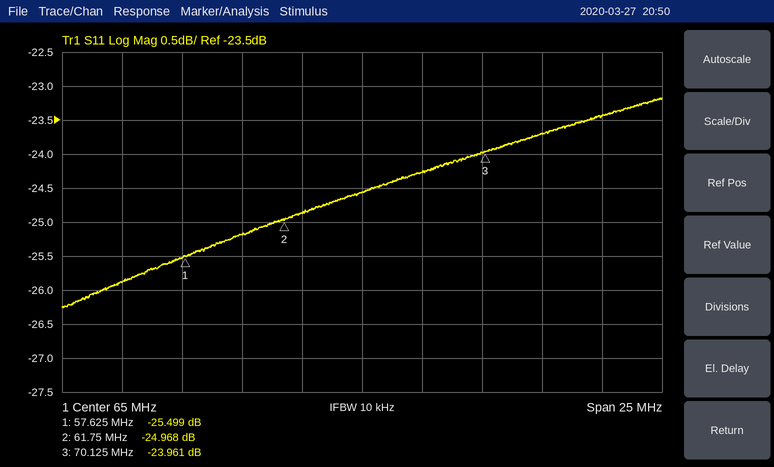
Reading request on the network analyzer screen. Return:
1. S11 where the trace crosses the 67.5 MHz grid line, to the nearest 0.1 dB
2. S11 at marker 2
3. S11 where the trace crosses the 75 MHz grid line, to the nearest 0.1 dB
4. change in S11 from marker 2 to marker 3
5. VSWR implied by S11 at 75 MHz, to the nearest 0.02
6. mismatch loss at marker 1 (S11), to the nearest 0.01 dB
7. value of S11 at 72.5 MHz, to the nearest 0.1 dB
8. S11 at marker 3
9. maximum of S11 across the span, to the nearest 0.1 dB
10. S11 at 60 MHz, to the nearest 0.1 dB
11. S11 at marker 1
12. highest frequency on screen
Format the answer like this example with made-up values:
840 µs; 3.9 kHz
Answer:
-24.3 dB; -24.968 dB; -23.4 dB; 1.007 dB; 1.14; 0.01 dB; -23.7 dB; -23.961 dB; -23.2 dB; -25.2 dB; -25.499 dB; 77.5 MHz
